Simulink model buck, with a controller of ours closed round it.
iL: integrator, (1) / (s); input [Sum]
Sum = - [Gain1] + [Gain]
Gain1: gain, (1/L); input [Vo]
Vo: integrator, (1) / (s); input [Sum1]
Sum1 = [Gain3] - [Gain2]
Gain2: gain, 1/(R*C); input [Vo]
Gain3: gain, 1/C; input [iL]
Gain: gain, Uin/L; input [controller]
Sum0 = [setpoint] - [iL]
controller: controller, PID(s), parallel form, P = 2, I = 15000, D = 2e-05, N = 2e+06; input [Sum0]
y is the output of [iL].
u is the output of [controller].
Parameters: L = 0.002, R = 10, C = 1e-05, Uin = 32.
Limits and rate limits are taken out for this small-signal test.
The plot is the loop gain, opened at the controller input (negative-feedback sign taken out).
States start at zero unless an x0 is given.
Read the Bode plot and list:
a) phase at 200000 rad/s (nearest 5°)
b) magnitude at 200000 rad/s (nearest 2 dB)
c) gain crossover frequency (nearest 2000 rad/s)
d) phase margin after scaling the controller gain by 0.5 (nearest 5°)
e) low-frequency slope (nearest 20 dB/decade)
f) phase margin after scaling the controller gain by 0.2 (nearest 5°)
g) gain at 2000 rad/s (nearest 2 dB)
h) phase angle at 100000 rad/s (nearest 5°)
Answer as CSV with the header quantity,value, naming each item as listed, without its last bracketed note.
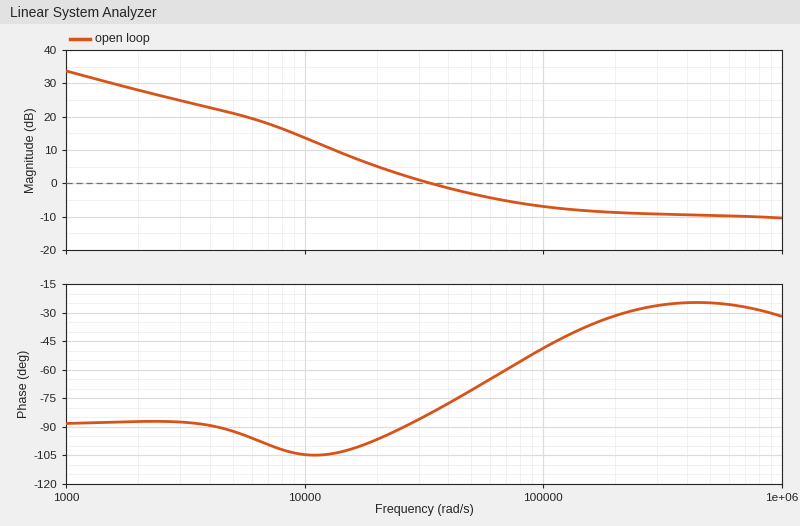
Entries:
quantity,value
phase at 200000 rad/s,-30°
magnitude at 200000 rad/s,-8 dB
gain crossover frequency,34000 rad/s
phase margin after scaling the controller gain by 0.5,80°
low-frequency slope,-20 dB/decade
phase margin after scaling the controller gain by 0.2,75°
gain at 2000 rad/s,28 dB
phase angle at 100000 rad/s,-50°
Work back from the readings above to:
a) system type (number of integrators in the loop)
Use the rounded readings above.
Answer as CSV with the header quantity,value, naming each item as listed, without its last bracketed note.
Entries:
quantity,value
system type,1
